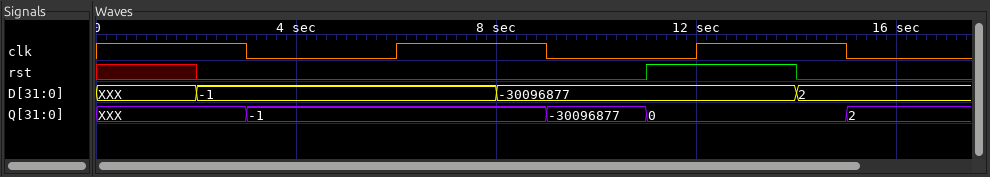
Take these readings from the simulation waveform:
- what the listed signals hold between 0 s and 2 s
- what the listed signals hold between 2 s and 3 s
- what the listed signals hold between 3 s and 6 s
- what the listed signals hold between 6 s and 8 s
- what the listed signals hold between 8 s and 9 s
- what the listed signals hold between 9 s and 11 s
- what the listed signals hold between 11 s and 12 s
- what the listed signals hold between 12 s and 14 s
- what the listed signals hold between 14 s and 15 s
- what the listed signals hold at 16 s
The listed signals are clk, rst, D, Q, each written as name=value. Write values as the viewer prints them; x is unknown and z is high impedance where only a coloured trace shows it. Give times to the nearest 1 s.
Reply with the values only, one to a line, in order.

clk=1, rst=x, D=XXX, Q=XXX
clk=1, rst=0, D=-1, Q=XXX
clk=0, rst=0, D=-1, Q=-1
clk=1, rst=0, D=-1, Q=-1
clk=1, rst=0, D=-30096877, Q=-1
clk=0, rst=0, D=-30096877, Q=-30096877
clk=0, rst=1, D=-30096877, Q=0
clk=1, rst=1, D=-30096877, Q=0
clk=1, rst=0, D=2, Q=0
clk=0, rst=0, D=2, Q=2
